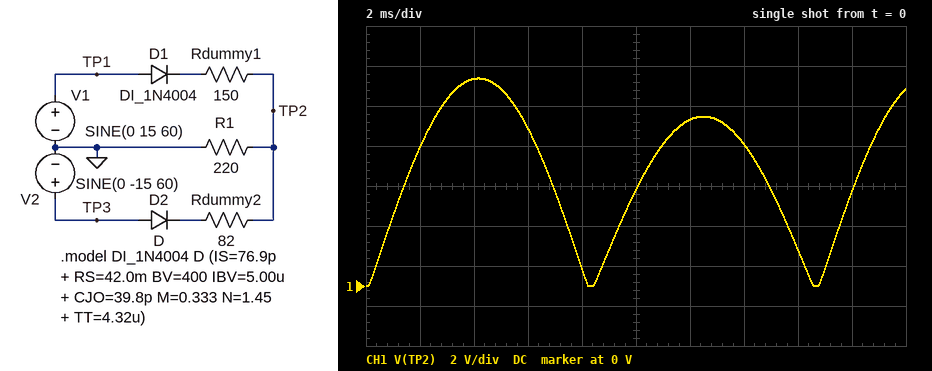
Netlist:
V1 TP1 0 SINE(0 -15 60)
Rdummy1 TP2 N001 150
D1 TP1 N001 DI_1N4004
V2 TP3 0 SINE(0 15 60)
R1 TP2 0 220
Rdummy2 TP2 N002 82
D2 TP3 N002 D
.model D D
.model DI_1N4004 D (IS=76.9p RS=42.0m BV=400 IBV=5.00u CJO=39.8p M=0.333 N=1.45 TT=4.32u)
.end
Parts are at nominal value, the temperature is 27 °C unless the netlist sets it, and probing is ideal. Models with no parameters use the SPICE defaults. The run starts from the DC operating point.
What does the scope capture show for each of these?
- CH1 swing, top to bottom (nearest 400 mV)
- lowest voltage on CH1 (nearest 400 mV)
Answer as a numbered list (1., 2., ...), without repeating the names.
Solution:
1. 10.4 V
2. 0 V
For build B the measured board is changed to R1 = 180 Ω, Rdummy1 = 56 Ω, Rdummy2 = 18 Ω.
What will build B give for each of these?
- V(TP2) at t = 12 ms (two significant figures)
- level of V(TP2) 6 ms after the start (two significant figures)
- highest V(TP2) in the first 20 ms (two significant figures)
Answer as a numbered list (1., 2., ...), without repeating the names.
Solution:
1. 11 V
2. 9.8 V
3. 13 V
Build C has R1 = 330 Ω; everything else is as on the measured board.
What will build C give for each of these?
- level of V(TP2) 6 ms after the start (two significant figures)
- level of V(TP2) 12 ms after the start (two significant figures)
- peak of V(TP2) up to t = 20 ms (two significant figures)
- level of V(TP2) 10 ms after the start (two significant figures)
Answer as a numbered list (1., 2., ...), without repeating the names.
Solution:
1. 8.7 V
2. 9.6 V
3. 11 V
4. 5.6 V
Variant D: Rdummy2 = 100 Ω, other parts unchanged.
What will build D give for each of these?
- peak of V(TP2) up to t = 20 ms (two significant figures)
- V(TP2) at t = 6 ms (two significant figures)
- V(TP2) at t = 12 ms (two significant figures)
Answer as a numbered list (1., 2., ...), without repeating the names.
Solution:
1. 9.8 V
2. 7.4 V
3. 8.3 V
